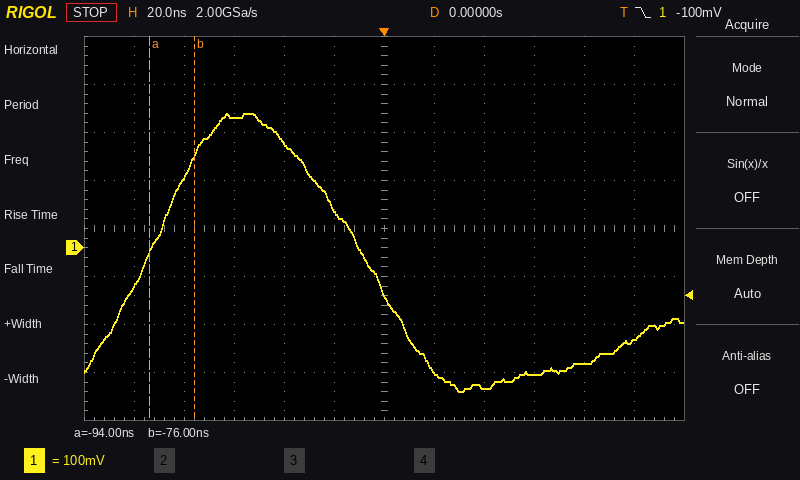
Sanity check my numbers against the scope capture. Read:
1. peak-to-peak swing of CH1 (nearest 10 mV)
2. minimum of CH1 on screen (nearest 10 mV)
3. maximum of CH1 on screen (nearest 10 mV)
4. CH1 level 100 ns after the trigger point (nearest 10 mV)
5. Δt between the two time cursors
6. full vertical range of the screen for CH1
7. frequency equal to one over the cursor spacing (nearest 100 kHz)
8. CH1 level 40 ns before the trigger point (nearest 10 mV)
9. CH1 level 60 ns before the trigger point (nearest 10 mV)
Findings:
580 mV
-300 mV
280 mV
-190 mV
18 ns
800 mV
55.6 MHz
220 mV
270 mV
